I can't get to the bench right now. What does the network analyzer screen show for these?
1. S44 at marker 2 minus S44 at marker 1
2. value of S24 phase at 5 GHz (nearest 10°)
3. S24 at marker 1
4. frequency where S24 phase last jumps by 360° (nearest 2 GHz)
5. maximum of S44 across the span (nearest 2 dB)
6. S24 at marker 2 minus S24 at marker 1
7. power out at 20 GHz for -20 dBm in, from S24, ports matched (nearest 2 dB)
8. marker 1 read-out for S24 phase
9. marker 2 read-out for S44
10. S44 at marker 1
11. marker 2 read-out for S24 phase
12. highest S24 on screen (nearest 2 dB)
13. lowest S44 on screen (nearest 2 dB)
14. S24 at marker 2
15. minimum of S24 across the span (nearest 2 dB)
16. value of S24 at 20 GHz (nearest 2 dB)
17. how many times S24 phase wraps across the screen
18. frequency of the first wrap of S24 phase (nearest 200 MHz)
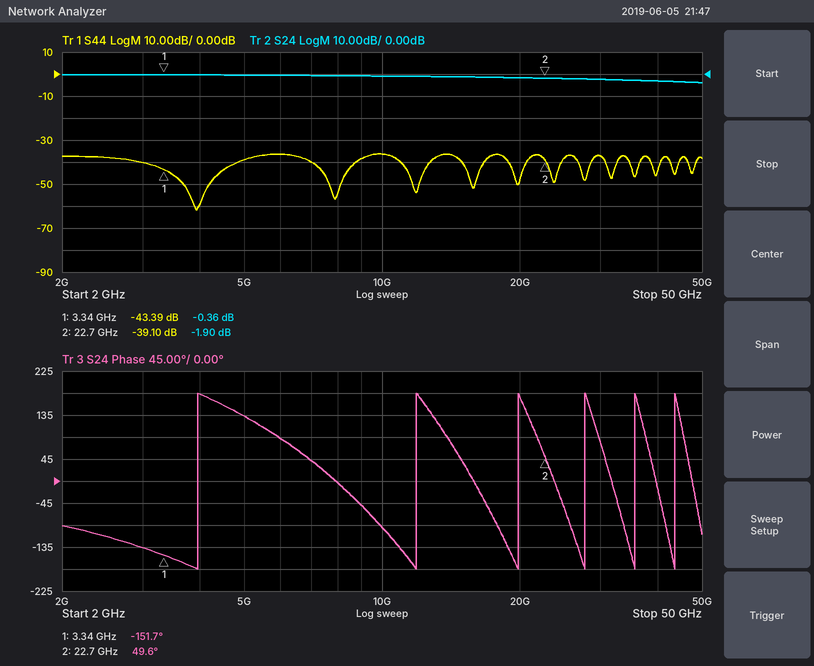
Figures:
4.29 dB
130°
-0.36 dB
44 GHz
-36 dB
-1.54 dB
-22 dBm
-151.7°
-39.10 dB
-43.39 dB
49.6°
0 dB
-62 dB
-1.90 dB
-4 dB
-2 dB
6
4.0 GHz
